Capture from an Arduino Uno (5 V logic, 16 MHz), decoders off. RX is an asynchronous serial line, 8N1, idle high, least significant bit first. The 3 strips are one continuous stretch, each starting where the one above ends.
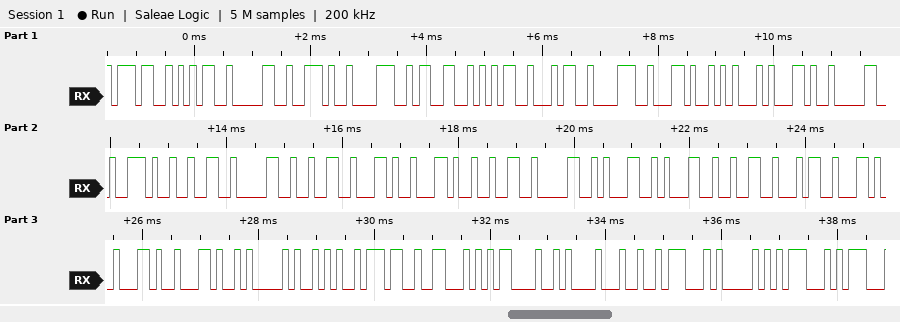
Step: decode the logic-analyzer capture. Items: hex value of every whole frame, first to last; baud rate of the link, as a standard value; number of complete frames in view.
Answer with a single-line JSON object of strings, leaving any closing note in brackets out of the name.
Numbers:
{"hex value of every whole frame, first to last": "37 35 30 2E 38 33 35 34 38 2C 45 2C 30 2E 32 30 32 2C 2C 32 30 31 31 32 34 2C 2C 2C 41 2A 37 46 0D 0A 24 47 50 47", "baud rate of the link, as a standard value": "9600 baud", "number of complete frames in view": "38"}
